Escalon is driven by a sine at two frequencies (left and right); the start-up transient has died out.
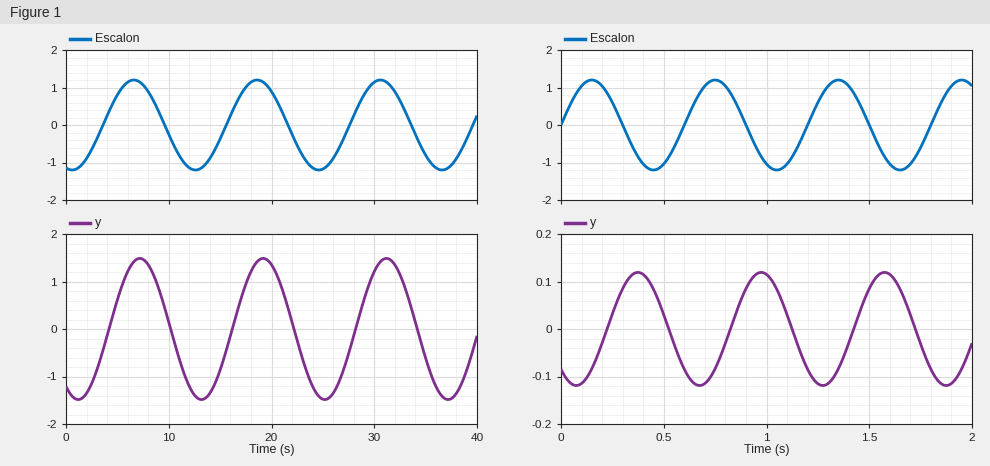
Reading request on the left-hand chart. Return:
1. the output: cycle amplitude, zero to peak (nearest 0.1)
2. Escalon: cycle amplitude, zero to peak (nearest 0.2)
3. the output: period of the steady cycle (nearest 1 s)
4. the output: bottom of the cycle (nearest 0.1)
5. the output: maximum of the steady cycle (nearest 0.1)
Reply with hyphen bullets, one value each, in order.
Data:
- 1.5
- 1.2
- 12 s
- -1.5
- 1.5
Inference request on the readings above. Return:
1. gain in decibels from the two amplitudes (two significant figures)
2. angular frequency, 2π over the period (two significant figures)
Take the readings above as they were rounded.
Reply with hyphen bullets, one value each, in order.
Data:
- 1.9 dB
- 0.52 rad/s
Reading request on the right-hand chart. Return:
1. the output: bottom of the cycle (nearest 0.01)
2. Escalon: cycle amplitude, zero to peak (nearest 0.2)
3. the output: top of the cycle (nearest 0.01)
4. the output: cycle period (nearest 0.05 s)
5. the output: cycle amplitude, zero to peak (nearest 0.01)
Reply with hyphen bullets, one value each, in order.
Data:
- -0.12
- 1.2
- 0.12
- 0.60 s
- 0.12
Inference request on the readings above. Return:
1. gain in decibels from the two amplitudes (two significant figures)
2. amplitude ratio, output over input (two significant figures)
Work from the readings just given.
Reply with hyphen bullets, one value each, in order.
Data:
- -20 dB
- 0.10
